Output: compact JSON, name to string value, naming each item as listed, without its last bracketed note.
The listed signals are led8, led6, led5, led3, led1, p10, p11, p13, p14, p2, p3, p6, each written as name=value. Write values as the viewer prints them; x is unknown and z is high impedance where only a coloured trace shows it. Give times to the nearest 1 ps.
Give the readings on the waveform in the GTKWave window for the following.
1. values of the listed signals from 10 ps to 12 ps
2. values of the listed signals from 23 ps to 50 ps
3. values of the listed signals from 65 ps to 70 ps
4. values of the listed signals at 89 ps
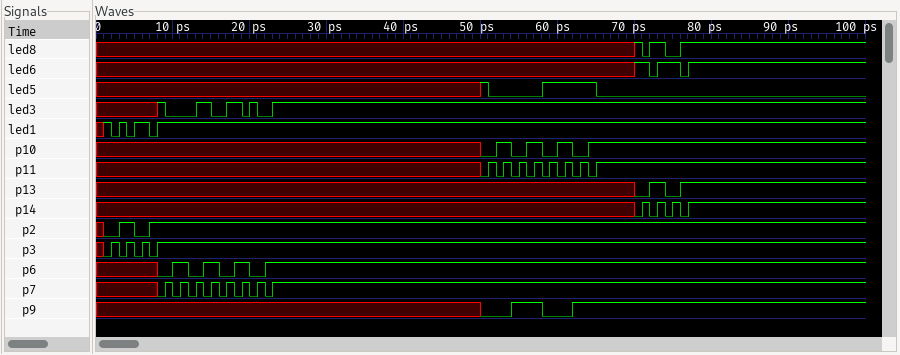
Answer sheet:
{"values of the listed signals from 10 ps to 12 ps": "led8=x, led6=x, led5=x, led3=0, led1=1, p10=x, p11=x, p13=x, p14=x, p2=1, p3=1, p6=1", "values of the listed signals from 23 ps to 50 ps": "led8=x, led6=x, led5=x, led3=1, led1=1, p10=x, p11=x, p13=x, p14=x, p2=1, p3=1, p6=1", "values of the listed signals from 65 ps to 70 ps": "led8=x, led6=x, led5=0, led3=1, led1=1, p10=1, p11=1, p13=x, p14=x, p2=1, p3=1, p6=1", "values of the listed signals at 89 ps": "led8=1, led6=1, led5=0, led3=1, led1=1, p10=1, p11=1, p13=1, p14=1, p2=1, p3=1, p6=1"}
